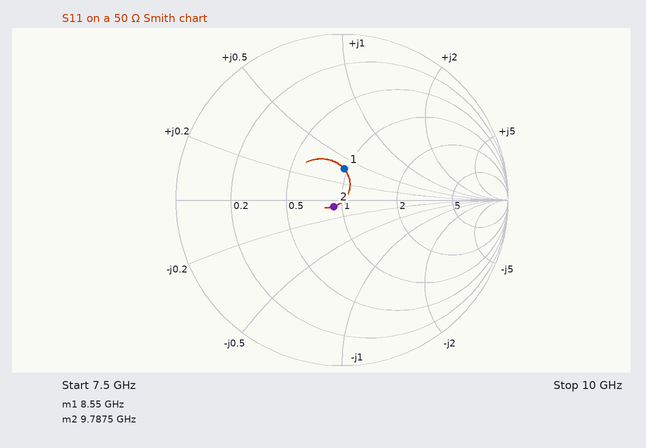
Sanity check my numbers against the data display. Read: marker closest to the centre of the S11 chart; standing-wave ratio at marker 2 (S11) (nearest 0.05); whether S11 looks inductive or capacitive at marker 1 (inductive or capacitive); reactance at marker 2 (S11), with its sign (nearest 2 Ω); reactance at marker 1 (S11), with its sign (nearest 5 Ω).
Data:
marker 2
1.15
inductive
-4 Ω
+20 Ω
